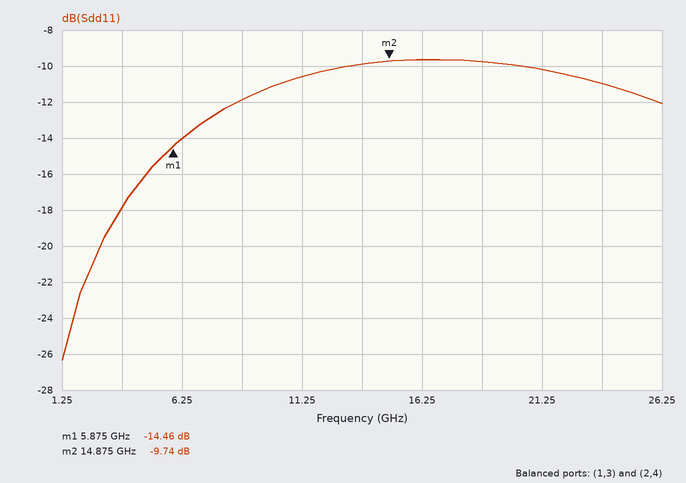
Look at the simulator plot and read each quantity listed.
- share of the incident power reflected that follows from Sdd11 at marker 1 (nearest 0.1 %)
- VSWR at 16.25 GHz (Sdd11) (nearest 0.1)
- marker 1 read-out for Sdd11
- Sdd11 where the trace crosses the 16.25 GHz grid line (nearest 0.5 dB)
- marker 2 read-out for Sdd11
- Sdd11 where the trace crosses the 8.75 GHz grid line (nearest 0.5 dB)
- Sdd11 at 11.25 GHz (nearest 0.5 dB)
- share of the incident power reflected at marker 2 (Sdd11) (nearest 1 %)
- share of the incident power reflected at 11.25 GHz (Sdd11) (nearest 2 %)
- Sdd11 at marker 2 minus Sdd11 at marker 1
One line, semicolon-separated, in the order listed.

3.6 %; 2.0; -14.46 dB; -9.5 dB; -9.74 dB; -12.0 dB; -10.5 dB; 11 %; 8 %; 4.72 dB
